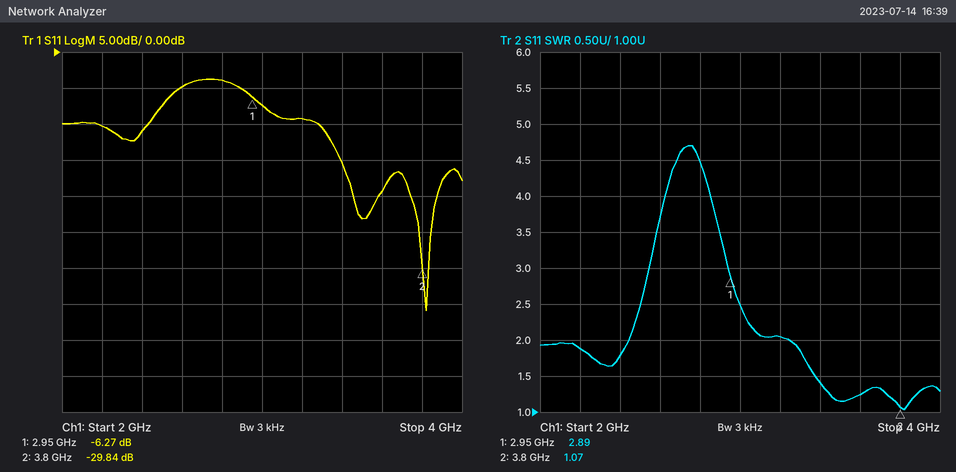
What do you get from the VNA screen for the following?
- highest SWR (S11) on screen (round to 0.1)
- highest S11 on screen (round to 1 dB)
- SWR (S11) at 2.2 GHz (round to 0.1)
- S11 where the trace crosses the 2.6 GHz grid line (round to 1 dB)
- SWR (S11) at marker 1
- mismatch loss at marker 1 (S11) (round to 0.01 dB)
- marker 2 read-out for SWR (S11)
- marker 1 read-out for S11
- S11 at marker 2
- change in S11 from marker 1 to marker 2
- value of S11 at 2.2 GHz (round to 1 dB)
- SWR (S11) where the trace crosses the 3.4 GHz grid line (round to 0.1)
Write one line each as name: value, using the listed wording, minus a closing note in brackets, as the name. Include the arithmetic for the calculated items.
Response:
highest SWR (S11) on screen: 4.7
highest S11 on screen: -4 dB
SWR (S11) at 2.2 GHz: 1.9
S11 where the trace crosses the 2.6 GHz grid line: -5 dB
SWR (S11) at marker 1: 2.89
mismatch loss at marker 1 (S11): −10 log10(1 − 10^(-6.27/10)) ≈ 1.17 dB
marker 2 read-out for SWR: 1.07
marker 1 read-out for S11: -6.27 dB
S11 at marker 2: -29.84 dB
change in S11 from marker 1 to marker 2: -29.84 − (-6.27) = -23.57 dB
value of S11 at 2.2 GHz: -10 dB
SWR (S11) where the trace crosses the 3.4 GHz grid line: 1.4
